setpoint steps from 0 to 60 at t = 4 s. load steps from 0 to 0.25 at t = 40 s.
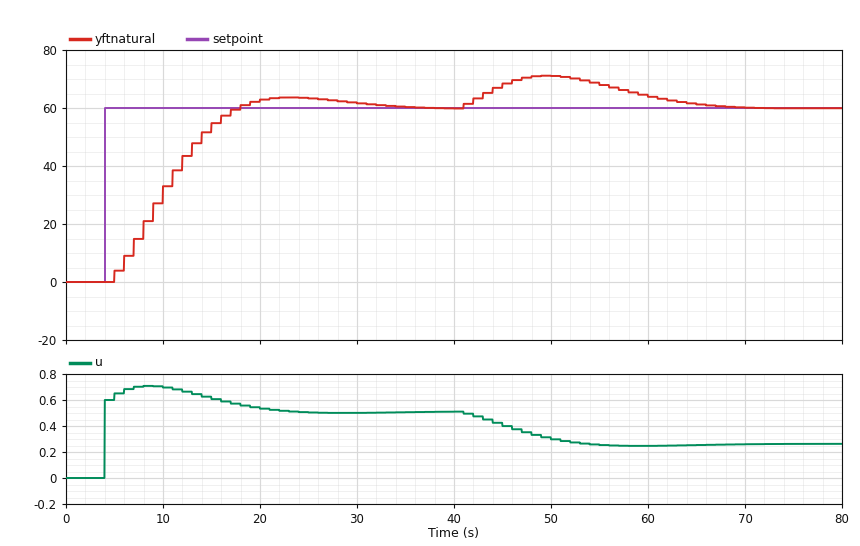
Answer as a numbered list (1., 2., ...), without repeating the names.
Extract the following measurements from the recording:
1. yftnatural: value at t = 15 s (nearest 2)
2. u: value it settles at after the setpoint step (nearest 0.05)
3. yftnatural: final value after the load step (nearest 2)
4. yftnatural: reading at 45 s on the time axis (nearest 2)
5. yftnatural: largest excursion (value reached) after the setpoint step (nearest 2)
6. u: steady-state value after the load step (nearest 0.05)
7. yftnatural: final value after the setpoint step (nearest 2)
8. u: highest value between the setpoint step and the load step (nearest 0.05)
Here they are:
1. 54
2. 0.50
3. 60
4. 68
5. 64
6. 0.25
7. 60
8. 0.70
